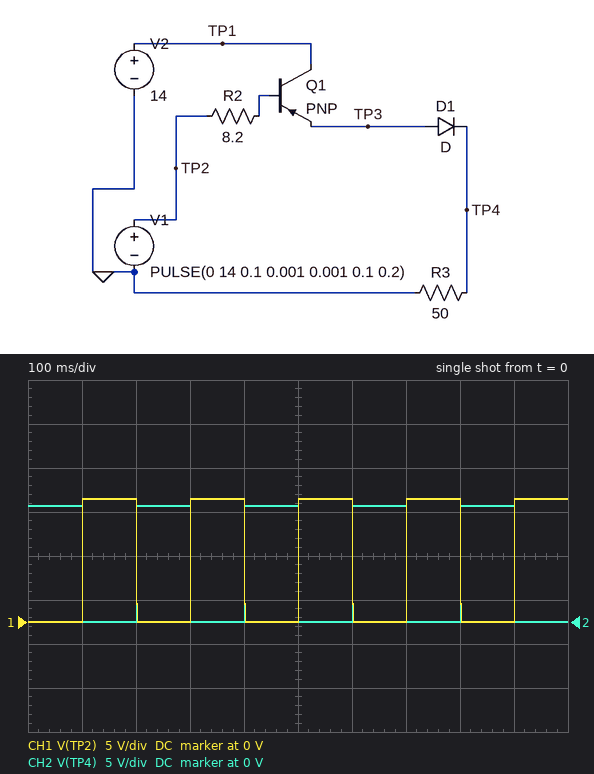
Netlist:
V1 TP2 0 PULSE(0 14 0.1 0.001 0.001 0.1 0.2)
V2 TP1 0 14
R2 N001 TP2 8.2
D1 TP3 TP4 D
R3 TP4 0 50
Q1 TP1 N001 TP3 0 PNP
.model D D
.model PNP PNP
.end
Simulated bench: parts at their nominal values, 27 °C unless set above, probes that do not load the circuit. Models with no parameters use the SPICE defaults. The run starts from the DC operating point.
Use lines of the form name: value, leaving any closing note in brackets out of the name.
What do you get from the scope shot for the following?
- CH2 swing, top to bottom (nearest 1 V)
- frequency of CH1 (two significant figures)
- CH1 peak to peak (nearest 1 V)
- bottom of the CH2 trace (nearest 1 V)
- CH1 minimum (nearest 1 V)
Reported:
CH2 swing, top to bottom: 13 V
frequency of CH1: 5.0 Hz
CH1 peak to peak: 14 V
bottom of the CH2 trace: 0 V
CH1 minimum: 0 V
